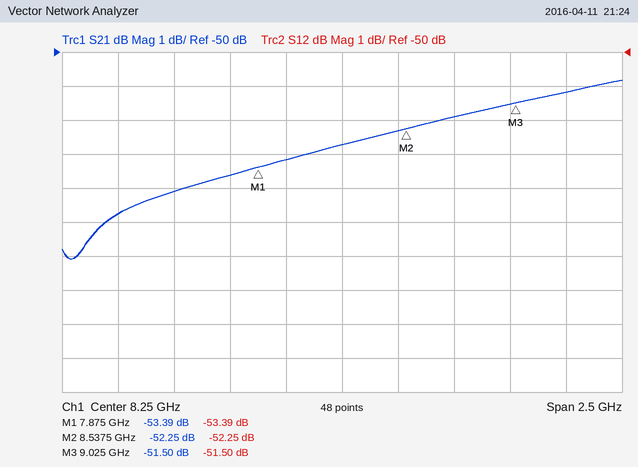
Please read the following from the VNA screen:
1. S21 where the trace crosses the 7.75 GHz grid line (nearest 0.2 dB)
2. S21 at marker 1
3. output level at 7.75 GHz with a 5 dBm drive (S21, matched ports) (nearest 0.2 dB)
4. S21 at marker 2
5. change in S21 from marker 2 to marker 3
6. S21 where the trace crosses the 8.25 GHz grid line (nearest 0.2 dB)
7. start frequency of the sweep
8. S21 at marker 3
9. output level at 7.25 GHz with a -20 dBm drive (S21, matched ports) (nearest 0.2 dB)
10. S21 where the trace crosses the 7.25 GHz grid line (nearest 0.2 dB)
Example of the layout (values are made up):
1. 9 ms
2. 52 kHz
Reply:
1. -53.6 dB
2. -53.39 dB
3. -48.6 dBm
4. -52.25 dB
5. 0.75 dB
6. -52.8 dB
7. 7 GHz
8. -51.50 dB
9. -74.8 dBm
10. -54.8 dB
